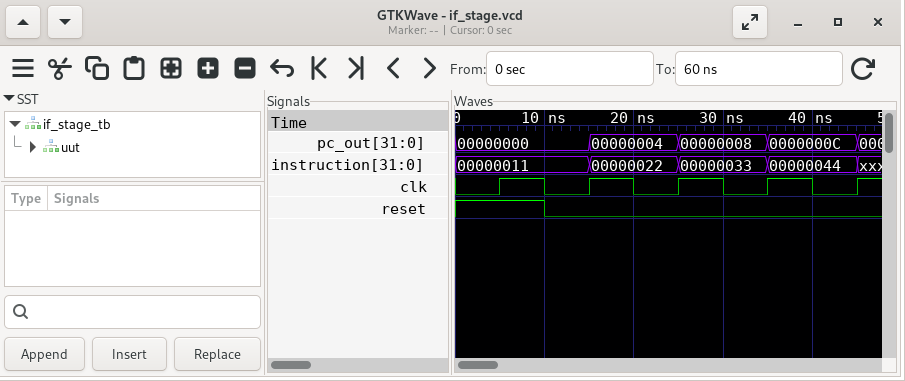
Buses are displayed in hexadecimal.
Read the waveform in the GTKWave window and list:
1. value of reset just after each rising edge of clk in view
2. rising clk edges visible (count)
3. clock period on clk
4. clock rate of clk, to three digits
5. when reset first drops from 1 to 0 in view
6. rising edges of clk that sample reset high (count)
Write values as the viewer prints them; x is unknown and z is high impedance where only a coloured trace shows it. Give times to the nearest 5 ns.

1 0 0 0 0
5
10 ns
100 MHz
10 ns
1
